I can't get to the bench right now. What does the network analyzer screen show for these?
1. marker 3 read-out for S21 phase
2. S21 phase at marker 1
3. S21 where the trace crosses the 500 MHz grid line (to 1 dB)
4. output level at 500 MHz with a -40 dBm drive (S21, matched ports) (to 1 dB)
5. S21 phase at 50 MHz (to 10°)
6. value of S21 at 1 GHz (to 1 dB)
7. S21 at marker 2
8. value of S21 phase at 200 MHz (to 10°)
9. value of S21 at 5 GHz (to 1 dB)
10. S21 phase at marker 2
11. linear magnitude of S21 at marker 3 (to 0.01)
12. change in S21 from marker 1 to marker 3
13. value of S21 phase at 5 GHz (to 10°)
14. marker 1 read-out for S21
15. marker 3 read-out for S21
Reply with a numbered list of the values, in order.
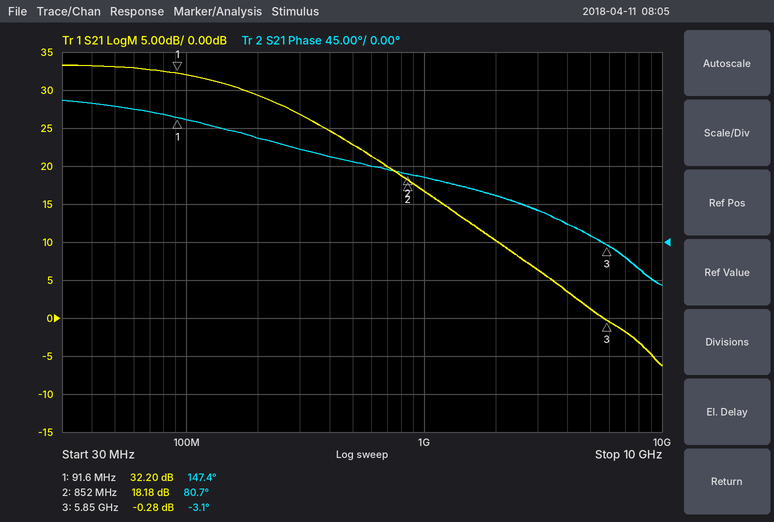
1. -3.1°
2. 147.4°
3. 23 dB
4. -17 dBm
5. 160°
6. 17 dB
7. 18.18 dB
8. 120°
9. 1 dB
10. 80.7°
11. 0.97
12. -32.48 dB
13. 10°
14. 32.20 dB
15. -0.28 dB
